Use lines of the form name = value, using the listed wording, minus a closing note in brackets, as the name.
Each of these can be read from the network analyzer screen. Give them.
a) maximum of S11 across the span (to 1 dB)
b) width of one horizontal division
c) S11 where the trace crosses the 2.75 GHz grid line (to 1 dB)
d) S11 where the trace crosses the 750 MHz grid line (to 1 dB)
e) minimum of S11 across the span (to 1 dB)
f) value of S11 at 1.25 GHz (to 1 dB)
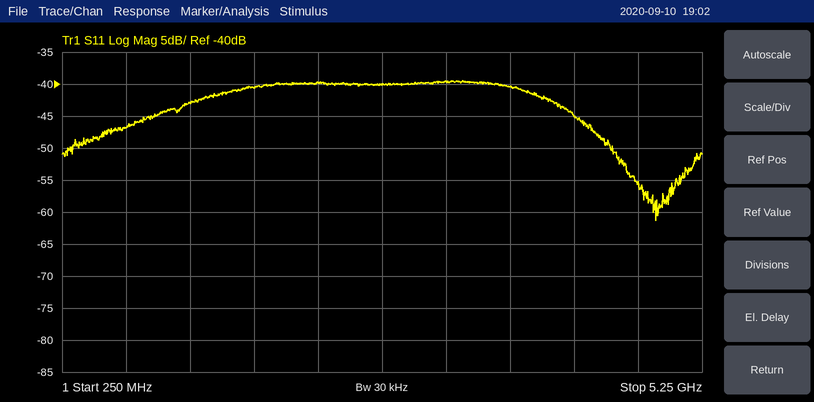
maximum of S11 across the span = -39 dB
width of one horizontal division = 500 MHz
S11 where the trace crosses the 2.75 GHz grid line = -40 dB
S11 where the trace crosses the 750 MHz grid line = -47 dB
minimum of S11 across the span = -61 dB
value of S11 at 1.25 GHz = -43 dB
